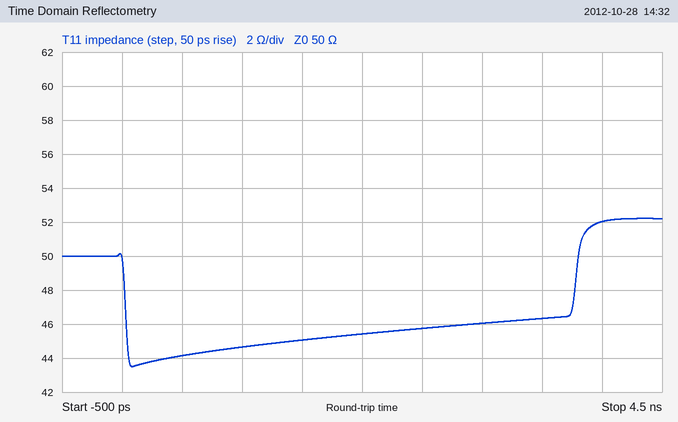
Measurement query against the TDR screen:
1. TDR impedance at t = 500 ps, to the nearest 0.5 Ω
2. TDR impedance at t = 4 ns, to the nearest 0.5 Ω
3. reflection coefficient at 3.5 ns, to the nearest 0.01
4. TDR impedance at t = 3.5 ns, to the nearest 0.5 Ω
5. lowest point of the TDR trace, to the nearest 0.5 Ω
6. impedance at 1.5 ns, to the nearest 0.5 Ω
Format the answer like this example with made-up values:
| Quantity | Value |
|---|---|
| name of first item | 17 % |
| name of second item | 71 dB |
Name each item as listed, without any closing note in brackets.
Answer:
| Quantity | Value |
|---|---|
| TDR impedance at t = 500 ps, to the nearest 0.5 Ω | 44.0 Ω |
| TDR impedance at t = 4 ns, to the nearest 0.5 Ω | 52.0 Ω |
| reflection coefficient at 3.5 ns, to the nearest 0.01 | -0.04 |
| TDR impedance at t = 3.5 ns, to the nearest 0.5 Ω | 46.5 Ω |
| lowest point of the TDR trace, to the nearest 0.5 Ω | 43.5 Ω |
| impedance at 1.5 ns, to the nearest 0.5 Ω | 45.0 Ω |
